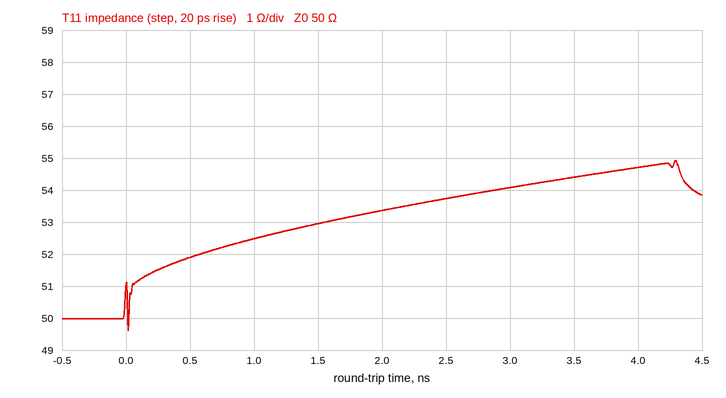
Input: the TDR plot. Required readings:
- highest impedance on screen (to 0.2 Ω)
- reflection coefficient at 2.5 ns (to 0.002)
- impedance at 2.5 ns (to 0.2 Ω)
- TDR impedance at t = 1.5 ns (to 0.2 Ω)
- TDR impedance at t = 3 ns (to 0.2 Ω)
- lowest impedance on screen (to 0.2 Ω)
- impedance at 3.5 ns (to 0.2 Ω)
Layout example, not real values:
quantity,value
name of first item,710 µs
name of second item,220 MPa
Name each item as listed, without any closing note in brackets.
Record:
quantity,value
highest impedance on screen,55.0 Ω
reflection coefficient at 2.5 ns,+0.036
impedance at 2.5 ns,53.8 Ω
TDR impedance at t = 1.5 ns,53.0 Ω
TDR impedance at t = 3 ns,54.0 Ω
lowest impedance on screen,49.6 Ω
impedance at 3.5 ns,54.4 Ω
